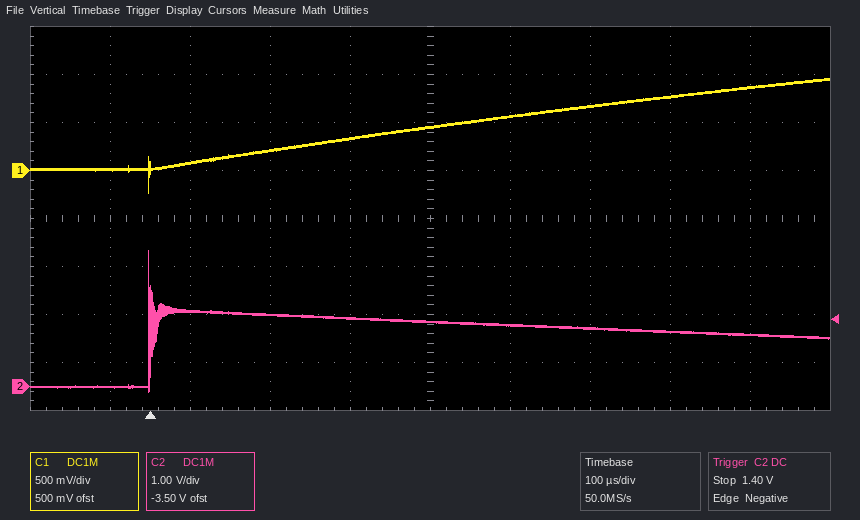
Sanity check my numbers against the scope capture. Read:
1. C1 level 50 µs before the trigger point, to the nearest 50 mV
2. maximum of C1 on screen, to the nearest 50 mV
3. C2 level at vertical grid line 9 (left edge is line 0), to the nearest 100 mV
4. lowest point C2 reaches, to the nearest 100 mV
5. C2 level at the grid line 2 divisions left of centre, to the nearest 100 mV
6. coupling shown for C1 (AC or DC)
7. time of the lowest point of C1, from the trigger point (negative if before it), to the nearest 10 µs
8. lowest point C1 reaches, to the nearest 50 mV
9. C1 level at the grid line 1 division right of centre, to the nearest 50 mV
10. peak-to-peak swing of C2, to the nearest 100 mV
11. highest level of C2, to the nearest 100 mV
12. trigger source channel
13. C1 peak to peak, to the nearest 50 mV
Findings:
0 mV
950 mV
1.1 V
-100 mV
1.5 V
DC
0 µs
-250 mV
550 mV
2.9 V
2.8 V
C2
1.20 V
